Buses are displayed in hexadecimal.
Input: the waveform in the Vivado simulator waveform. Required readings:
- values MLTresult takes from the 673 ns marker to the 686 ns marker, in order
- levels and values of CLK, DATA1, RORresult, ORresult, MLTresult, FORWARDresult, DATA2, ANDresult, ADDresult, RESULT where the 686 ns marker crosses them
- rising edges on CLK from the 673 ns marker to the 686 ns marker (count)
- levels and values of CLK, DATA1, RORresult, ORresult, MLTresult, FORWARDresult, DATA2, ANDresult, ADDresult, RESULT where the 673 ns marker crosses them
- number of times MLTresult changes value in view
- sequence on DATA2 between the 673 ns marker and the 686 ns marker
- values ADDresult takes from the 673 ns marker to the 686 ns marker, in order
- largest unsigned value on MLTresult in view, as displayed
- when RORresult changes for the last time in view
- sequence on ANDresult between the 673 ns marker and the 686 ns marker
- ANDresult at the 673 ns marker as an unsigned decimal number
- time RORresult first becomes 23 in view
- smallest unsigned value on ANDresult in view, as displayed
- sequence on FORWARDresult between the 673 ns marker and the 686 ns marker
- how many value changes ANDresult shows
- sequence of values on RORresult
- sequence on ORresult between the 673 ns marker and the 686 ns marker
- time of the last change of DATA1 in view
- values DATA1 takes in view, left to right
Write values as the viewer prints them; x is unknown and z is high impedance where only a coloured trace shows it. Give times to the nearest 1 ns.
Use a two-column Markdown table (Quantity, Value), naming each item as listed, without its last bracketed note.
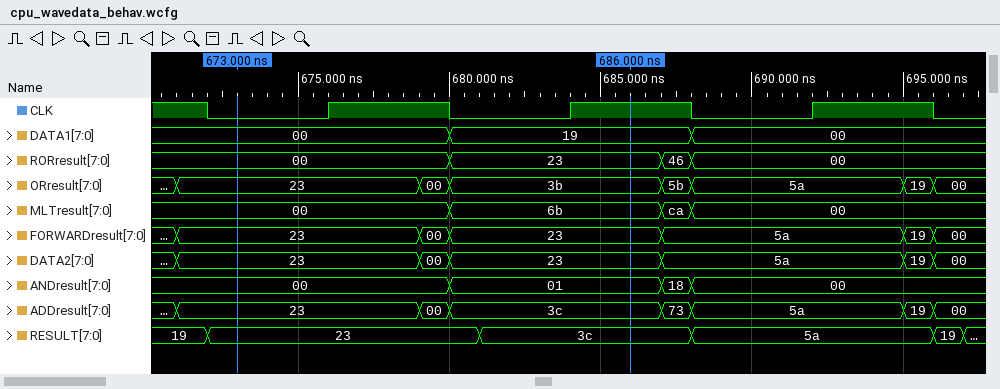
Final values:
| Quantity | Value |
|---|---|
| values MLTresult takes from the 673 ns marker to the 686 ns marker, in order | 00, 6b |
| levels and values of CLK, DATA1, RORresult, ORresult, MLTresult, FORWARDresult, DATA2, ANDresult, ADDresult, RESULT where the 686 ns marker crosses them | CLK=1, DATA1=19, RORresult=23, ORresult=3b, MLTresult=6b, FORWARDresult=23, DATA2=23, ANDresult=01, ADDresult=3c, RESULT=3c |
| rising edges on CLK from the 673 ns marker to the 686 ns marker | 2 |
| levels and values of CLK, DATA1, RORresult, ORresult, MLTresult, FORWARDresult, DATA2, ANDresult, ADDresult, RESULT where the 673 ns marker crosses them | CLK=0, DATA1=00, RORresult=00, ORresult=23, MLTresult=00, FORWARDresult=23, DATA2=23, ANDresult=00, ADDresult=23, RESULT=23 |
| number of times MLTresult changes value in view | 3 |
| sequence on DATA2 between the 673 ns marker and the 686 ns marker | 23, 00, 23 |
| values ADDresult takes from the 673 ns marker to the 686 ns marker, in order | 23, 00, 3c |
| largest unsigned value on MLTresult in view, as displayed | ca |
| when RORresult changes for the last time in view | 688 ns |
| sequence on ANDresult between the 673 ns marker and the 686 ns marker | 00, 01 |
| ANDresult at the 673 ns marker as an unsigned decimal number | 0 |
| time RORresult first becomes 23 in view | 680 ns |
| smallest unsigned value on ANDresult in view, as displayed | 00 |
| sequence on FORWARDresult between the 673 ns marker and the 686 ns marker | 23, 00, 23 |
| how many value changes ANDresult shows | 3 |
| sequence of values on RORresult | 00, 23, 46, 00 |
| sequence on ORresult between the 673 ns marker and the 686 ns marker | 23, 00, 3b |
| time of the last change of DATA1 in view | 688 ns |
| values DATA1 takes in view, left to right | 00, 19, 00 |
